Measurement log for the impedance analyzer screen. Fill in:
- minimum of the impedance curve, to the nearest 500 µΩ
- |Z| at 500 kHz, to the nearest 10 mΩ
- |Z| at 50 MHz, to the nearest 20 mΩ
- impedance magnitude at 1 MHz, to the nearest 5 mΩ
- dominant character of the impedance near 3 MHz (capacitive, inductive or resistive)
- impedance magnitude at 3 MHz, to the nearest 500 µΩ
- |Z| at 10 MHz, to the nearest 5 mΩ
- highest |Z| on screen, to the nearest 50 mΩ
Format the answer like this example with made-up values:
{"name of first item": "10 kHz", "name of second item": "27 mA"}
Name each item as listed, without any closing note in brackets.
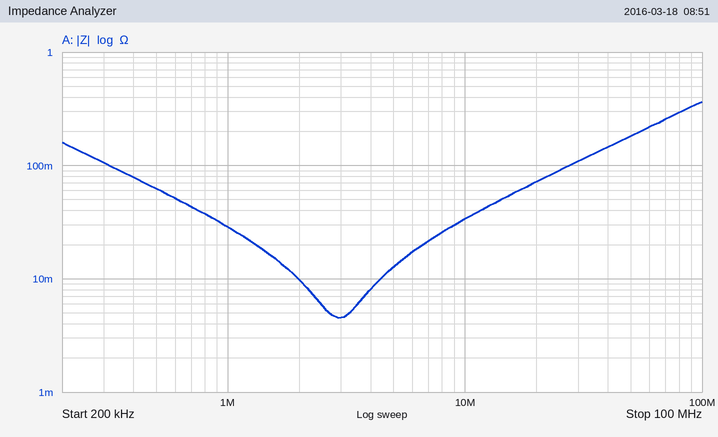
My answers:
{"minimum of the impedance curve, to the nearest 500 µΩ": "4.5 mΩ", "|Z| at 500 kHz, to the nearest 10 mΩ": "60 mΩ", "|Z| at 50 MHz, to the nearest 20 mΩ": "180 mΩ", "impedance magnitude at 1 MHz, to the nearest 5 mΩ": "30 mΩ", "dominant character of the impedance near 3 MHz": "resistive", "impedance magnitude at 3 MHz, to the nearest 500 µΩ": "4.5 mΩ", "|Z| at 10 MHz, to the nearest 5 mΩ": "35 mΩ", "highest |Z| on screen, to the nearest 50 mΩ": "350 mΩ"}
